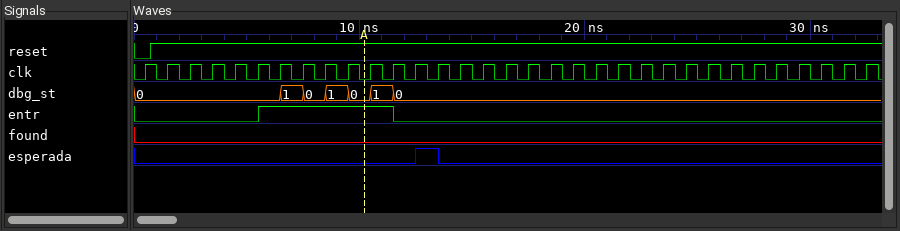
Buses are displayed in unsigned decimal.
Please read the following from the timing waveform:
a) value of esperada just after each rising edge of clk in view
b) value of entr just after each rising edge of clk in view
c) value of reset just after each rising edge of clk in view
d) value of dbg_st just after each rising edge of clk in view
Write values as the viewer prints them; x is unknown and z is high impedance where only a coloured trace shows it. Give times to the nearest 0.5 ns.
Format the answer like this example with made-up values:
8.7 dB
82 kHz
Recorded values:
0 0 0 0 0 0 0 0 0 0 0 0 1 0 0 0 0 0 0 0 0 0 0 0 0 0 0 0 0 0 0 0 0
0 0 0 0 0 1 1 1 1 1 1 0 0 0 0 0 0 0 0 0 0 0 0 0 0 0 0 0 0 0 0 0 0
0 1 1 1 1 1 1 1 1 1 1 1 1 1 1 1 1 1 1 1 1 1 1 1 1 1 1 1 1 1 1 1 1
0, 0, 0, 0, 0, 0, 1, 0, 1, 0, 1, 0, 0, 0, 0, 0, 0, 0, 0, 0, 0, 0, 0, 0, 0, 0, 0, 0, 0, 0, 0, 0, 0
